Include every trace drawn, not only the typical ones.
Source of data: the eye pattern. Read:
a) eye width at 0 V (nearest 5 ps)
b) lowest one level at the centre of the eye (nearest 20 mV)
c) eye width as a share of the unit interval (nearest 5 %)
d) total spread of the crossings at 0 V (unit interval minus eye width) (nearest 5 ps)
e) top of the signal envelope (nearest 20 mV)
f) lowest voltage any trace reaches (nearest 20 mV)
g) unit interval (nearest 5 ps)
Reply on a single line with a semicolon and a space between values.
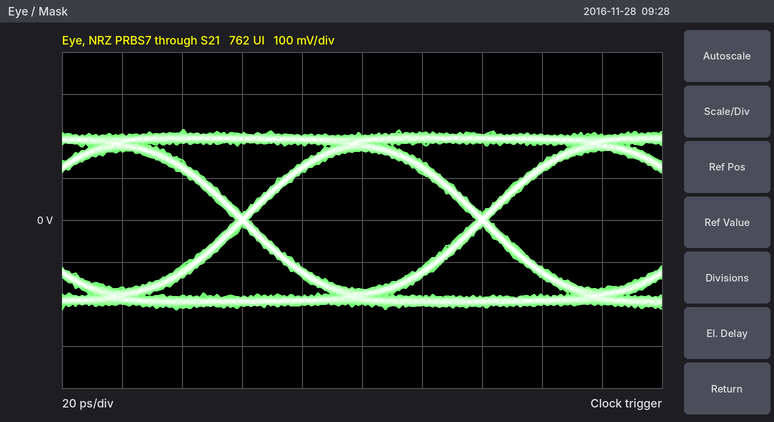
75 ps; 160 mV; 95 %; 5 ps; 220 mV; -220 mV; 80 ps
